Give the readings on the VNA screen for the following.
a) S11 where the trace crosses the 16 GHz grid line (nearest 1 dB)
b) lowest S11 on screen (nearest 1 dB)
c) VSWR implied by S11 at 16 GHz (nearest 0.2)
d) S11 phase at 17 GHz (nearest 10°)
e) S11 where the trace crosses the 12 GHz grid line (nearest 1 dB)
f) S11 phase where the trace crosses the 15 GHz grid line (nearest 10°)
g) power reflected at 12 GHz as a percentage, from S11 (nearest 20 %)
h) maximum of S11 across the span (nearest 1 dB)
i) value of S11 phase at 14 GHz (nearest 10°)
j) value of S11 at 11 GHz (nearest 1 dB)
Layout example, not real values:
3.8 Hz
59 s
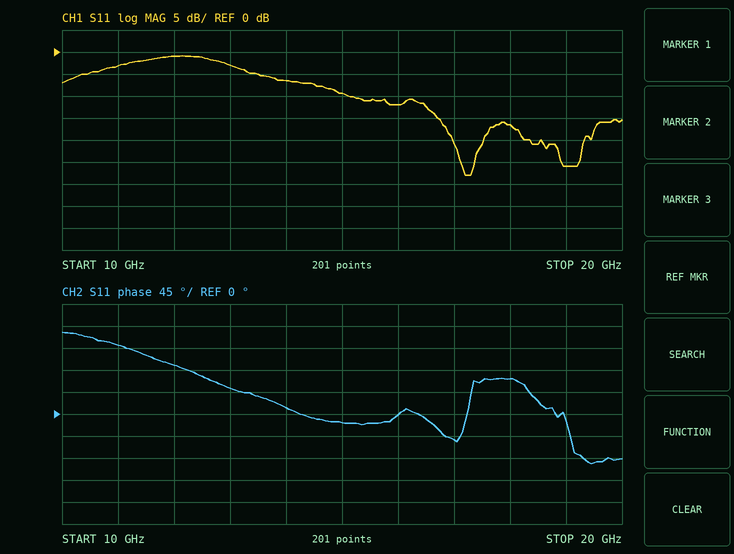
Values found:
-12 dB
-28 dB
1.6
-50°
-1 dB
-20°
80 %
-1 dB
10°
-3 dB
